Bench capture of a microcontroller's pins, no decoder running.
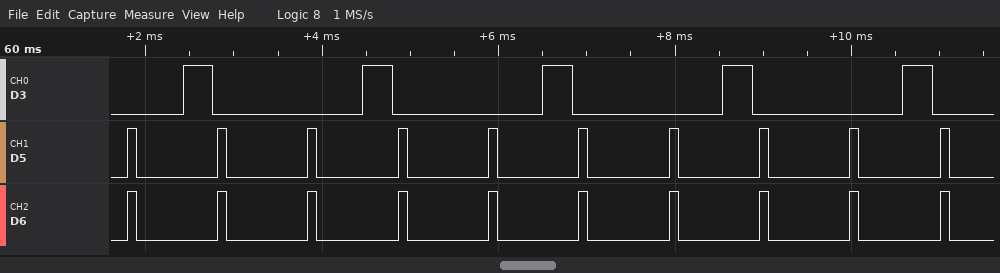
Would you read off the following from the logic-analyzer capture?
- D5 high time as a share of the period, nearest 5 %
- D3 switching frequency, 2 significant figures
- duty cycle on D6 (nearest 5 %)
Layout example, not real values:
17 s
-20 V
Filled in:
10 %
490 Hz
10 %
